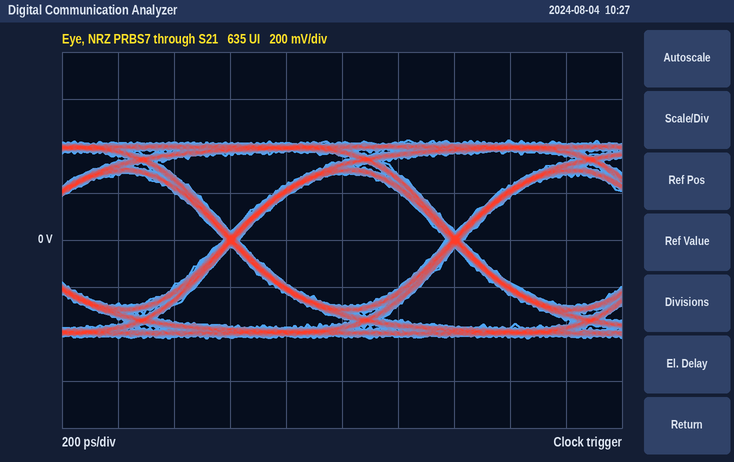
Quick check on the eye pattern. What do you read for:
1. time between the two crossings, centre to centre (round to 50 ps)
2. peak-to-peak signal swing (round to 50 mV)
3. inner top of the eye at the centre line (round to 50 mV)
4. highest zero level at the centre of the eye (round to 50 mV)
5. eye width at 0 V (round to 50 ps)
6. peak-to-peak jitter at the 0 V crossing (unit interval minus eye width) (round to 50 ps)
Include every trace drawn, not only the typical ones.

800 ps
850 mV
300 mV
-300 mV
750 ps
50 ps
